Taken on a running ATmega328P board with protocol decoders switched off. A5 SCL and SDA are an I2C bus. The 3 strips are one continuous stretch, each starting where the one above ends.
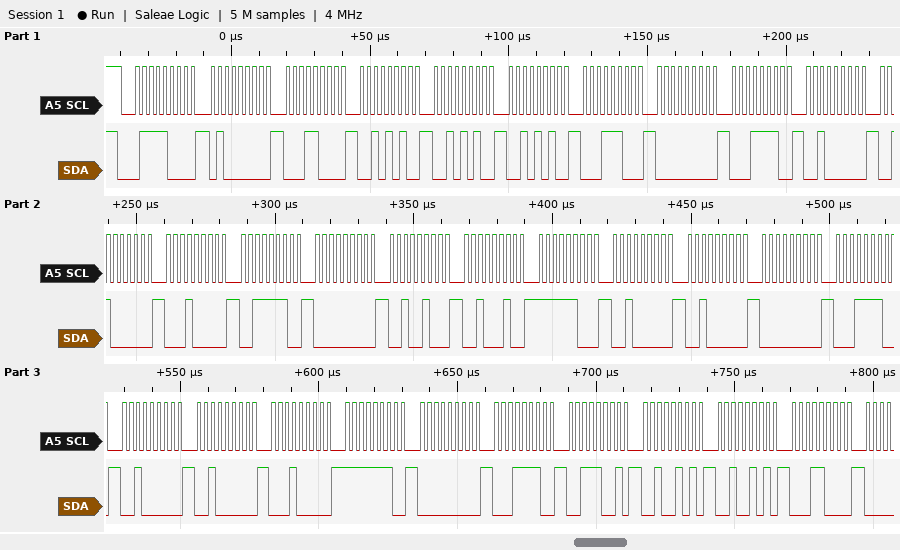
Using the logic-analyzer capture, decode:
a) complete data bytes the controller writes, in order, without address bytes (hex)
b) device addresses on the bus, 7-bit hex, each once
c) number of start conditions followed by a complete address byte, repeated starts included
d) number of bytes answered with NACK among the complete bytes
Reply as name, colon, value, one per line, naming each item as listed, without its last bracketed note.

complete data bytes the controller writes, in order, without address bytes: 40 18 2A 2A 2A 1C 00 1E 20 20 10 3E 00 24 22 FC 20 20 00 1E 20 20 10 FE 00 1E 39 25 25 18
device addresses on the bus, 7-bit hex, each once: 0x3C
number of start conditions followed by a complete address byte, repeated starts included: 1
number of bytes answered with NACK among the complete bytes: 0
